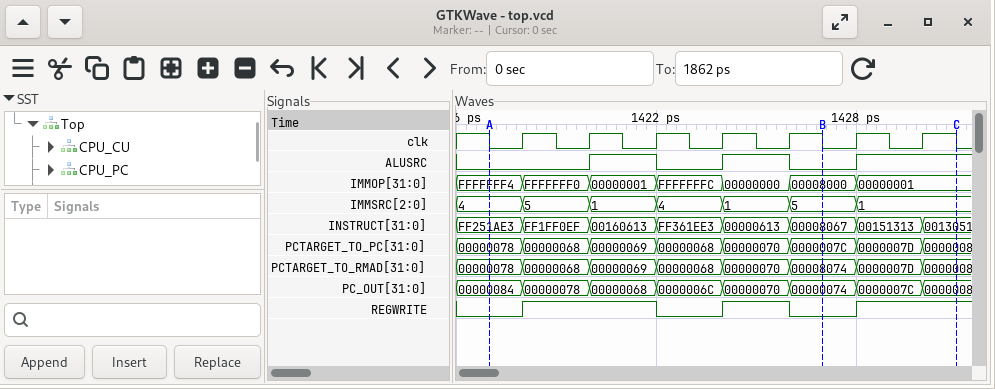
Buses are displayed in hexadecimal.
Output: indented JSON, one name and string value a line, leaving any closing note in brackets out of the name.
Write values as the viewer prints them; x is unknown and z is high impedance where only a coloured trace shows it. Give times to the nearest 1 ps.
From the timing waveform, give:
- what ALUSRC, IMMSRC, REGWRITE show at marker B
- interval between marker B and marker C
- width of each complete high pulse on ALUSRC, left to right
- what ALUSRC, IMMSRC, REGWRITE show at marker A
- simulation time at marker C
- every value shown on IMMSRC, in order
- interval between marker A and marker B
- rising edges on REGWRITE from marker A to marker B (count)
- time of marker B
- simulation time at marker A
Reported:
{
  "what ALUSRC, IMMSRC, REGWRITE show at marker B": "ALUSRC=0, IMMSRC=5, REGWRITE=0",
  "interval between marker B and marker C": "4 ps",
  "width of each complete high pulse on ALUSRC, left to right": "2 ps, 2 ps",
  "what ALUSRC, IMMSRC, REGWRITE show at marker A": "ALUSRC=0, IMMSRC=4, REGWRITE=0",
  "simulation time at marker C": "1431 ps",
  "every value shown on IMMSRC, in order": "4, 5, 1, 4, 1, 5, 1",
  "interval between marker A and marker B": "10 ps",
  "rising edges on REGWRITE from marker A to marker B": "2",
  "time of marker B": "1427 ps",
  "simulation time at marker A": "1417 ps"
}
